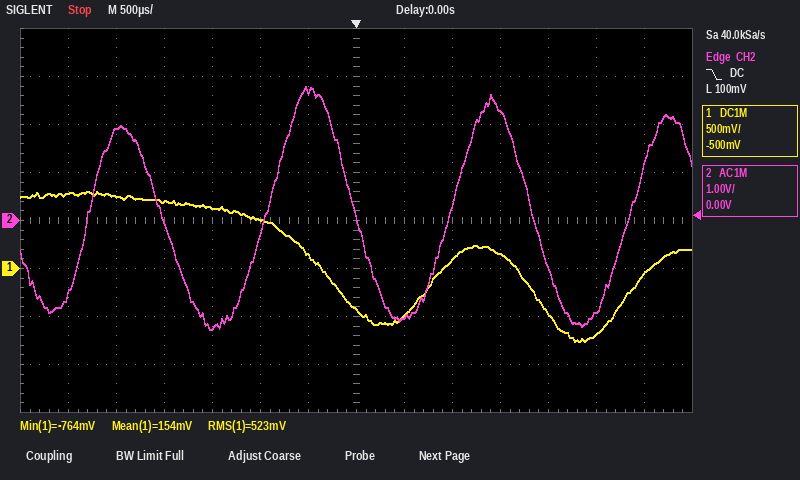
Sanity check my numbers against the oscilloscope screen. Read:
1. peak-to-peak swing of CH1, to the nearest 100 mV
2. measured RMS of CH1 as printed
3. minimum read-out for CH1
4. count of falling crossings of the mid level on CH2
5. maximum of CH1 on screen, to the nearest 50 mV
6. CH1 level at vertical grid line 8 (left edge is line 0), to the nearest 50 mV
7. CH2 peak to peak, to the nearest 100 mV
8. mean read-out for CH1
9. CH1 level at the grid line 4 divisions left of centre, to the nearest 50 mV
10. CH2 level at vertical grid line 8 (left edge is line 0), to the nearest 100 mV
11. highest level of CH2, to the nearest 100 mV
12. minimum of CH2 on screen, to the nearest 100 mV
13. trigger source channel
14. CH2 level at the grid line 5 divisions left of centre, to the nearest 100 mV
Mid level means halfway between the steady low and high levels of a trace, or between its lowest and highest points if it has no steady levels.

1.60 V
523 mV
-764 mV
3
800 mV
-500 mV
5.1 V
154 mV
700 mV
-2.0 V
2.8 V
-2.3 V
CH2
1.9 V
